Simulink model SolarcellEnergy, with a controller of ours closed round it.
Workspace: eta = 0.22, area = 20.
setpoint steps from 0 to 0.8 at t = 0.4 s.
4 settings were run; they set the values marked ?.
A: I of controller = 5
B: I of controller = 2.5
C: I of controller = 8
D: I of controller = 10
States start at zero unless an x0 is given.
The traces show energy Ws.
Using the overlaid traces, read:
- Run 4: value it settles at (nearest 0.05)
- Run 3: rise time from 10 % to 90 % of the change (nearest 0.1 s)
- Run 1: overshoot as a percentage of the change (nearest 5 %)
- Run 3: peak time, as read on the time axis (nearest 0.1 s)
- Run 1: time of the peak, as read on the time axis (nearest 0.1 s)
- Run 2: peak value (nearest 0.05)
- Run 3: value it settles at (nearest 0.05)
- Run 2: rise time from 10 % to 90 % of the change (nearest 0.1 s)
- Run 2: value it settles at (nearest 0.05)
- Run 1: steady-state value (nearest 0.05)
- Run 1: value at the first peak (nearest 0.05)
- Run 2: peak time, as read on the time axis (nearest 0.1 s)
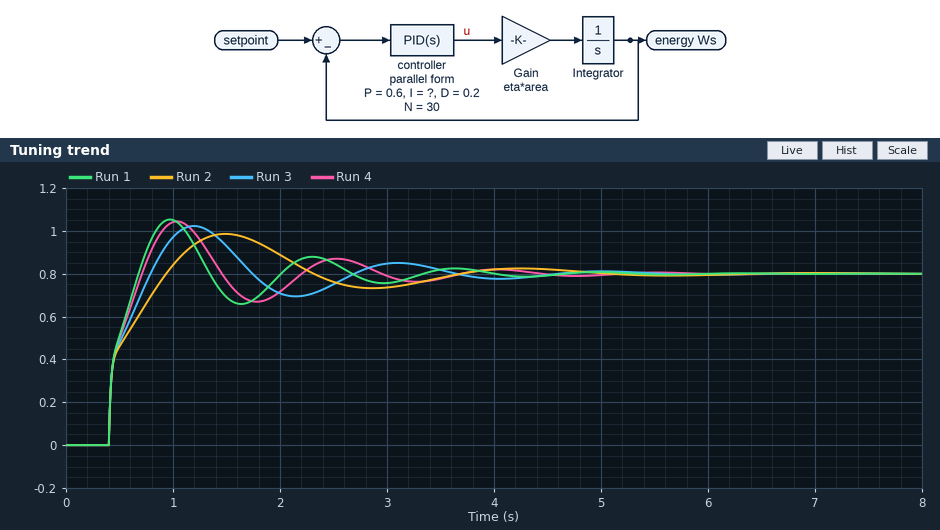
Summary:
0.80
0.3 s
30 %
1.2 s
1.0 s
1.00
0.80
0.4 s
0.80
0.80
1.05
1.5 s
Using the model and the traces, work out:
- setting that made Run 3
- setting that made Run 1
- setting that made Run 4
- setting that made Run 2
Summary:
A
D
C
B
